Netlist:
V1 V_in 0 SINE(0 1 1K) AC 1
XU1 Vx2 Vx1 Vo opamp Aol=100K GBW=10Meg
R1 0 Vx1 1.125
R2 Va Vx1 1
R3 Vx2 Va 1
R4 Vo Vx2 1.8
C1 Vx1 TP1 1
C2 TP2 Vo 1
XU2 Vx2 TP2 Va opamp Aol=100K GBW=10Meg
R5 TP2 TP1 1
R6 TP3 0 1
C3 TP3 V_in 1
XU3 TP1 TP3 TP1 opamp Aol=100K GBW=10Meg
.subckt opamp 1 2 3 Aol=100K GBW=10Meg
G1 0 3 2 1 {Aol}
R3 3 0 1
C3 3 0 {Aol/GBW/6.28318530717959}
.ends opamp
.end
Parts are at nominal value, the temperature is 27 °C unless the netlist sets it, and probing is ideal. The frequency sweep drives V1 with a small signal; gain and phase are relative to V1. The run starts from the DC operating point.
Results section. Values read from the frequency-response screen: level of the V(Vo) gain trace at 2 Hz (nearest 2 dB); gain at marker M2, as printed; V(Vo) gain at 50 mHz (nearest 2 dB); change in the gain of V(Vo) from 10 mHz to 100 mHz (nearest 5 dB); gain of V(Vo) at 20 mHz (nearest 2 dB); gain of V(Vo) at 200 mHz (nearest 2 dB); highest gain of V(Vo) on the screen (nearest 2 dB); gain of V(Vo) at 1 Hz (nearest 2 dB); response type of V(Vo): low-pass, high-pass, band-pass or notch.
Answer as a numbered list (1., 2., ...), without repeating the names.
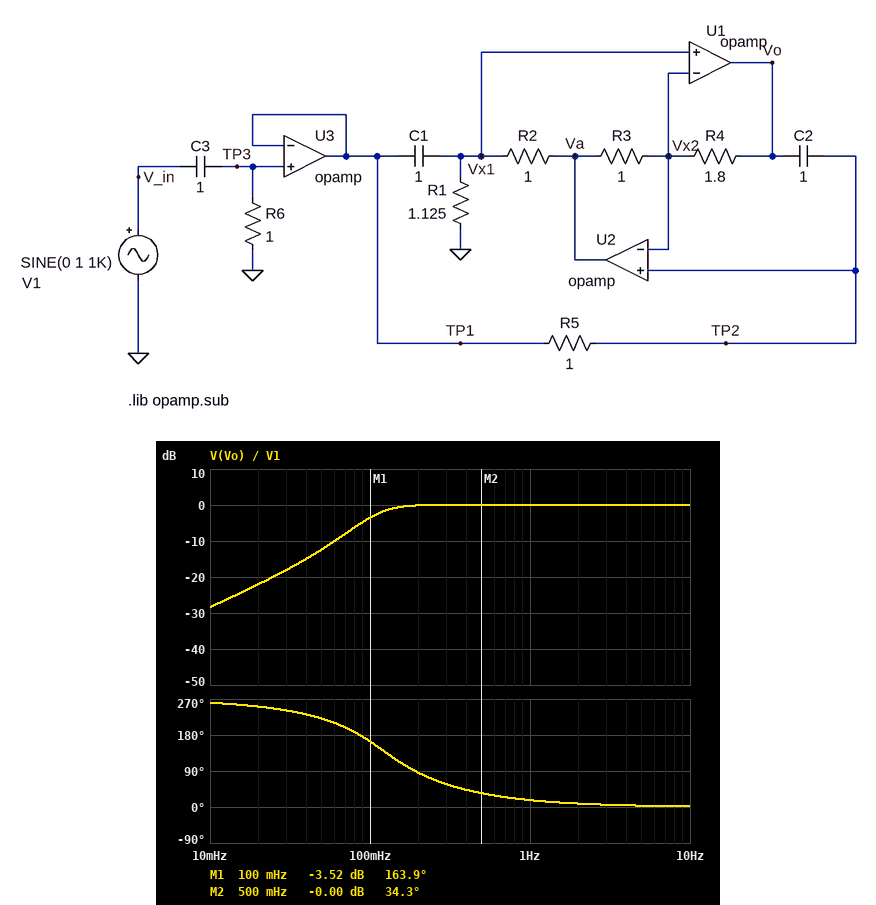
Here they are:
1. 0 dB
2. -0.00 dB
3. -12 dB
4. 25 dB
5. -22 dB
6. 0 dB
7. 0 dB
8. 0 dB
9. high-pass
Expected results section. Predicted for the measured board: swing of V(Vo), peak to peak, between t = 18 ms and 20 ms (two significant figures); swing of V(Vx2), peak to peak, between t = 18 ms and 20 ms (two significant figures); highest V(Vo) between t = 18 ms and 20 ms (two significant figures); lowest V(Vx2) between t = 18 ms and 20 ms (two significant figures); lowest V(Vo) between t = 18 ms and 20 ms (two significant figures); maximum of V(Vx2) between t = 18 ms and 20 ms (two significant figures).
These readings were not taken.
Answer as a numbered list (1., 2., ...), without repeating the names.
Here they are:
1. 2.0 V
2. 2.0 V
3. 1.0 V
4. -1.0 V
5. -1.0 V
6. 1.0 V
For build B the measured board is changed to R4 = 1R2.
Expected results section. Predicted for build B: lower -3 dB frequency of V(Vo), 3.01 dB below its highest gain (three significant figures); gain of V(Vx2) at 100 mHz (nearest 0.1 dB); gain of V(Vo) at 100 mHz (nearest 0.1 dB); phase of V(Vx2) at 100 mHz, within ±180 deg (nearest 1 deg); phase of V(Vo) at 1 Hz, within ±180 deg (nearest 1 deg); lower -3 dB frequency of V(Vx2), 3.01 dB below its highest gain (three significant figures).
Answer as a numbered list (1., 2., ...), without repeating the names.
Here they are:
1. 141 mHz
2. -9.7 dB
3. -9.4 dB
4. 6 deg
5. 17 deg
6. 276 mHz
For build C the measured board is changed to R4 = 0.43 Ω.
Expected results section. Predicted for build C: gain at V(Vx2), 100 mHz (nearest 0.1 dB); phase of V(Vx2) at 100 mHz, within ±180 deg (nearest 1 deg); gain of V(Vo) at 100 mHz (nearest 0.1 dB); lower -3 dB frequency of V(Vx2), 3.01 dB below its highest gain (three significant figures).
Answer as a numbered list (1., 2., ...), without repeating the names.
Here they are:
1. -5.8 dB
2. 42 deg
3. -11.2 dB
4. 346 mHz
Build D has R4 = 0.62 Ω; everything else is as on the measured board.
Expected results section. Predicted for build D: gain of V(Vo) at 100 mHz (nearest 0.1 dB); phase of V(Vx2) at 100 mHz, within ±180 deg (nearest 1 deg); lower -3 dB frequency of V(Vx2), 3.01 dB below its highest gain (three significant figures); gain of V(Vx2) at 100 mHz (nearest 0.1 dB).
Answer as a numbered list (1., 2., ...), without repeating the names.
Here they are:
1. -17.7 dB
2. 33 deg
3. 314 mHz
4. -6.3 dB
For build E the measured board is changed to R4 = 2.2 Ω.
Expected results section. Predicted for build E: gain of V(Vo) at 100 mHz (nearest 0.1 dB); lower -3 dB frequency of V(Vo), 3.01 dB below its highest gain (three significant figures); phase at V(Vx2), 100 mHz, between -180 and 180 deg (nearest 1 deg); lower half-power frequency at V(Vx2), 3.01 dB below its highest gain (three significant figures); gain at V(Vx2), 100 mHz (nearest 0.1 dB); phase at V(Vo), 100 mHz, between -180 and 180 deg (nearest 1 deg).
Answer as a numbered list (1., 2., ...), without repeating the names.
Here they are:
1. -2.1 dB
2. 89.2 mHz
3. -26 deg
4. 257 mHz
5. -24.9 dB
6. 154 deg
